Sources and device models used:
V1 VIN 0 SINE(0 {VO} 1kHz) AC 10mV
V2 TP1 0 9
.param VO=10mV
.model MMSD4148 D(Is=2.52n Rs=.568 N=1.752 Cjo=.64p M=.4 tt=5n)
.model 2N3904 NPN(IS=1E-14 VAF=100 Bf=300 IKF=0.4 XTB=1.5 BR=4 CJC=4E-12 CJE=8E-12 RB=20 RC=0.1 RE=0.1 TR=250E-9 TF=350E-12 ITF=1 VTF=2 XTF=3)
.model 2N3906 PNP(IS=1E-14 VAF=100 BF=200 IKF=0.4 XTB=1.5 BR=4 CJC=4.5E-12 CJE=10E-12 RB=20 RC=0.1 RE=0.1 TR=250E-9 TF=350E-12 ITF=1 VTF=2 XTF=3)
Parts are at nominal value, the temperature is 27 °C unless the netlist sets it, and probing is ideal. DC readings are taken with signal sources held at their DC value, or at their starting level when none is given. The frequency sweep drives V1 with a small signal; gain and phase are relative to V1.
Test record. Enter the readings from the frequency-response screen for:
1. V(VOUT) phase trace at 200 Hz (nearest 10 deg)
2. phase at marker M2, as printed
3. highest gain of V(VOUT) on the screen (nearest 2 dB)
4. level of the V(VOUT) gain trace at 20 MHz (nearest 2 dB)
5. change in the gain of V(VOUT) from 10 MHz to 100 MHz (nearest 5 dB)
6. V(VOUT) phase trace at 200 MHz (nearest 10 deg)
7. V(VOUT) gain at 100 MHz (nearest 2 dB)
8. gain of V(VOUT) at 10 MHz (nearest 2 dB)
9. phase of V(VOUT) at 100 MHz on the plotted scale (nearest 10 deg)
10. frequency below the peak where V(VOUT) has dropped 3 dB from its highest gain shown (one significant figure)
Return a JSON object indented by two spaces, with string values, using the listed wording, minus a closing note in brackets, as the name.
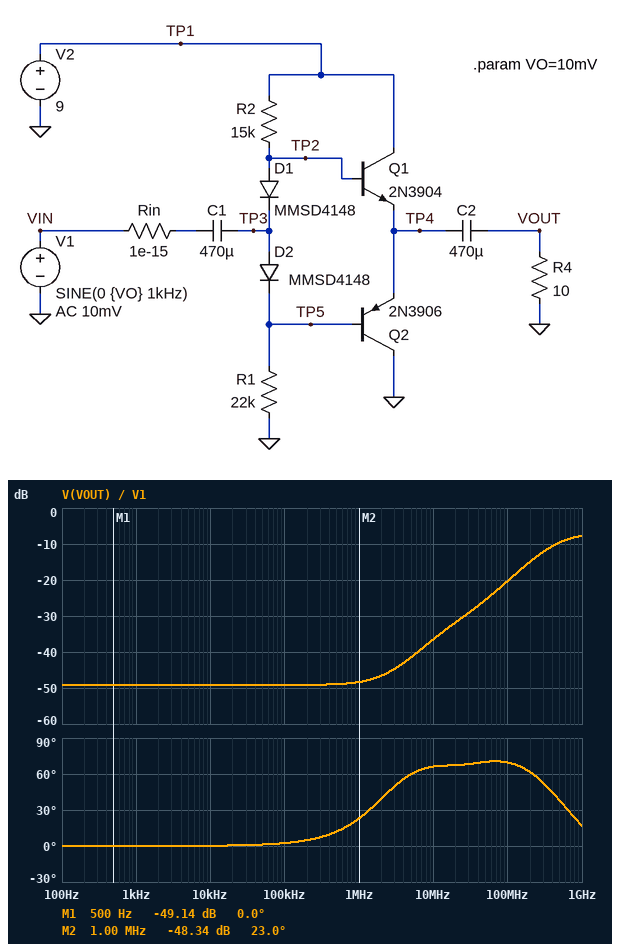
{
  "V(VOUT) phase trace at 200 Hz": "0 deg",
  "phase at marker M2, as printed": "23.0 deg",
  "highest gain of V(VOUT) on the screen": "-8 dB",
  "level of the V(VOUT) gain trace at 20 MHz": "-32 dB",
  "change in the gain of V(VOUT) from 10 MHz to 100 MHz": "15 dB",
  "V(VOUT) phase trace at 200 MHz": "60 deg",
  "V(VOUT) gain at 100 MHz": "-20 dB",
  "gain of V(VOUT) at 10 MHz": "-36 dB",
  "phase of V(VOUT) at 100 MHz on the plotted scale": "70 deg",
  "frequency below the peak where V(VOUT) has dropped 3 dB from its highest gain shown": "400 MHz"
}
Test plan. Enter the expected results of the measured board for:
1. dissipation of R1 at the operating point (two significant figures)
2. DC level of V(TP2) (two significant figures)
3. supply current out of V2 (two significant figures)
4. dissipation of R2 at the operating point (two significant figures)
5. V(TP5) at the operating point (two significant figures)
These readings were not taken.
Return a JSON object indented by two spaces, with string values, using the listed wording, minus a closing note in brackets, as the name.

{
  "dissipation of R1 at the operating point": "1.0 mW",
  "DC level of V(TP2)": "5.8 V",
  "supply current out of V2": "220 µA",
  "dissipation of R2 at the operating point": "700 µW",
  "V(TP5) at the operating point": "4.7 V"
}
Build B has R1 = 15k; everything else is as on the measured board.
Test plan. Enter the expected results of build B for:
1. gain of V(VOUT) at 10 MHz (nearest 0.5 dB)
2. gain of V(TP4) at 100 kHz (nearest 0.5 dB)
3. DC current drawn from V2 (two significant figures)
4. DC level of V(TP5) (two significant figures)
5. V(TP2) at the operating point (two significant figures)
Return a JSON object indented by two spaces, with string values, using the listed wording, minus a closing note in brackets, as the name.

{
  "gain of V(VOUT) at 10 MHz": "-36.0 dB",
  "gain of V(TP4) at 100 kHz": "-46.0 dB",
  "DC current drawn from V2": "270 µA",
  "DC level of V(TP5)": "4.0 V",
  "V(TP2) at the operating point": "5.0 V"
}
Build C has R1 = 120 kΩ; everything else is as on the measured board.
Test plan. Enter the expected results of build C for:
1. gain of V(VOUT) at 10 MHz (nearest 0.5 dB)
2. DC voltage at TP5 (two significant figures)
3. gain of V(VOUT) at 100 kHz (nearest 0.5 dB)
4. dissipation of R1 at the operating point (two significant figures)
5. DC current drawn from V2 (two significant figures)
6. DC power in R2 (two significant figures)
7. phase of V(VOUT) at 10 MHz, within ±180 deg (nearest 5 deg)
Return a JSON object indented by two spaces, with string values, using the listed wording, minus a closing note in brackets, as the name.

{
  "gain of V(VOUT) at 10 MHz": "-39.5 dB",
  "DC voltage at TP5": "7.2 V",
  "gain of V(VOUT) at 100 kHz": "-68.0 dB",
  "dissipation of R1 at the operating point": "430 µW",
  "DC current drawn from V2": "60 µA",
  "DC power in R2": "54 µW",
  "phase of V(VOUT) at 10 MHz, within ±180 deg": "60 deg"
}
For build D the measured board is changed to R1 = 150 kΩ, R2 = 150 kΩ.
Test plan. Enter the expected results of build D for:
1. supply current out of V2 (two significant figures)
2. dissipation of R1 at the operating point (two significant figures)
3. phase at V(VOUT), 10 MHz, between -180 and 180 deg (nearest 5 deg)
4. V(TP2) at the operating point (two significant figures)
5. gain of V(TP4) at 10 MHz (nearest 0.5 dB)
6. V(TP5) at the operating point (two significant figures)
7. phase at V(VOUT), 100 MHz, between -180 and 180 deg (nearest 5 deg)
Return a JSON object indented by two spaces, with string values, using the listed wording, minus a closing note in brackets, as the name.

{
  "supply current out of V2": "27 µA",
  "dissipation of R1 at the operating point": "110 µW",
  "phase at V(VOUT), 10 MHz, between -180 and 180 deg": "50 deg",
  "V(TP2) at the operating point": "4.9 V",
  "gain of V(TP4) at 10 MHz": "-42.5 dB",
  "V(TP5) at the operating point": "4.1 V",
  "phase at V(VOUT), 100 MHz, between -180 and 180 deg": "75 deg"
}
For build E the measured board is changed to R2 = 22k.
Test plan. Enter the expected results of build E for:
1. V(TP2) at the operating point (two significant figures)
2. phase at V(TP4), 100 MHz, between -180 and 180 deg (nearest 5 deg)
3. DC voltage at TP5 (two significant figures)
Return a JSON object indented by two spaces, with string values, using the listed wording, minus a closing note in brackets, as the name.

{
  "V(TP2) at the operating point": "5.0 V",
  "phase at V(TP4), 100 MHz, between -180 and 180 deg": "70 deg",
  "DC voltage at TP5": "4.0 V"
}
